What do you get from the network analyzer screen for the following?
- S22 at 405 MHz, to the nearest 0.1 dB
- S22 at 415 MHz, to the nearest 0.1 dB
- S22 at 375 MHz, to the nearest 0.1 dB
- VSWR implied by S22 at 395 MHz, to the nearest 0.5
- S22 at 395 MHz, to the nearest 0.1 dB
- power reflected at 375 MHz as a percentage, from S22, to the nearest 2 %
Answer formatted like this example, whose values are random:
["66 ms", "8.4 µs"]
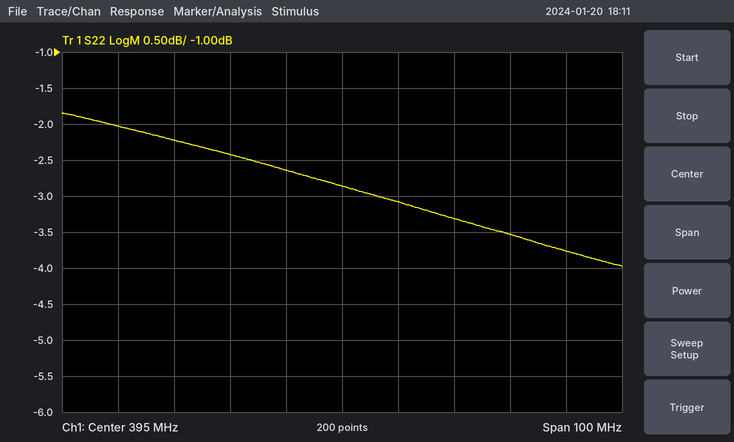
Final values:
["-3.1 dB", "-3.3 dB", "-2.4 dB", "6.0", "-2.9 dB", "58 %"]
